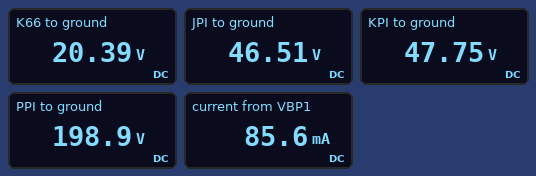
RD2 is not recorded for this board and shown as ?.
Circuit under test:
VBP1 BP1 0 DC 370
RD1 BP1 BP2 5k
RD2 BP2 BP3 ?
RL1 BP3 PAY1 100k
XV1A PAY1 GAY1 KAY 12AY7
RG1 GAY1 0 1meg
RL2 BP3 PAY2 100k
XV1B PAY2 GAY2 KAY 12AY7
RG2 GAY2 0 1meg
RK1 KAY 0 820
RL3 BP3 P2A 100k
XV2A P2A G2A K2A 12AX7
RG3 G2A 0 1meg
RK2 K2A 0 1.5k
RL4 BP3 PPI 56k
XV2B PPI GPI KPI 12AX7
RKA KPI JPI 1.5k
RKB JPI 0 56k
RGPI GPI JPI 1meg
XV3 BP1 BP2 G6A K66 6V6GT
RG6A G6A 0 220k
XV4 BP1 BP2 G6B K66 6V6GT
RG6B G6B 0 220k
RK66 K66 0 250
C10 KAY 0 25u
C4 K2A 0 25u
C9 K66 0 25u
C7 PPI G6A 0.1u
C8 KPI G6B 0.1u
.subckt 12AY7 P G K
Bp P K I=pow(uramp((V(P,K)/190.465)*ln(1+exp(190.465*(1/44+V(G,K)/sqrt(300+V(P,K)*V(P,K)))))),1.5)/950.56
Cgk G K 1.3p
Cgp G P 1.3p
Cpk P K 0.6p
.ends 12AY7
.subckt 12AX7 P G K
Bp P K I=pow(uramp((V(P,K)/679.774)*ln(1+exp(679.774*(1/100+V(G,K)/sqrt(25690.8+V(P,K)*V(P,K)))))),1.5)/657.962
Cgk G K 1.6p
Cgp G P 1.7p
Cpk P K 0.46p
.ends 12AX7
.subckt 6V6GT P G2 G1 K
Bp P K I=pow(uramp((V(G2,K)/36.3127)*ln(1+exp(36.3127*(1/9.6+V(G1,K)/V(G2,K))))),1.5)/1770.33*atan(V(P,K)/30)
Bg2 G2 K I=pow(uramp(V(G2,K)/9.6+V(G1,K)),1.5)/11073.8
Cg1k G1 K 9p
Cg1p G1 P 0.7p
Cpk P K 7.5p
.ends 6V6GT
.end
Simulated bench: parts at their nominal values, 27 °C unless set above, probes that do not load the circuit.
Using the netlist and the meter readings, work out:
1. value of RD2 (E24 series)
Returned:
18 kΩ
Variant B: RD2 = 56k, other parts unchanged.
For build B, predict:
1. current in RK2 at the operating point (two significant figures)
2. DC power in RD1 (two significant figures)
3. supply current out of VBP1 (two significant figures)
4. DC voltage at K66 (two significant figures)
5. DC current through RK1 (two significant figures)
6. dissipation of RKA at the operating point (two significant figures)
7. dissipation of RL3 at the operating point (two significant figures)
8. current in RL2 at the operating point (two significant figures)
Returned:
620 µA
420 mW
86 mA
21 V
1.6 mA
530 µW
38 mW
790 µA
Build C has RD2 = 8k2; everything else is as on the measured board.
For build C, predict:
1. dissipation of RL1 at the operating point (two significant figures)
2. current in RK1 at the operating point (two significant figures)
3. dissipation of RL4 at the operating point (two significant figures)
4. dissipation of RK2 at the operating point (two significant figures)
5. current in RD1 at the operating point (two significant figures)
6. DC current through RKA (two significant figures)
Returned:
180 mW
2.7 mA
48 mW
1.4 mW
11 mA
930 µA
